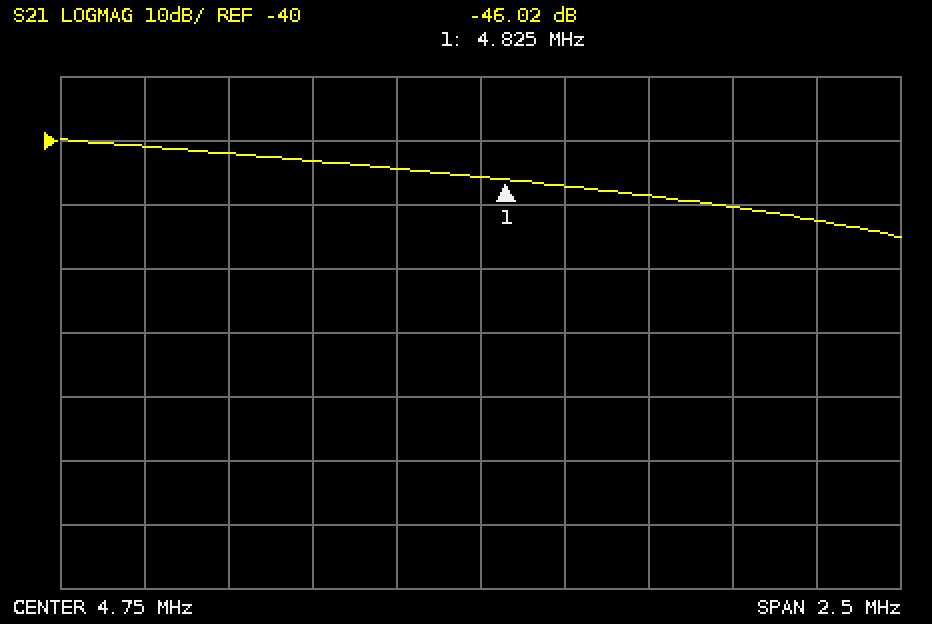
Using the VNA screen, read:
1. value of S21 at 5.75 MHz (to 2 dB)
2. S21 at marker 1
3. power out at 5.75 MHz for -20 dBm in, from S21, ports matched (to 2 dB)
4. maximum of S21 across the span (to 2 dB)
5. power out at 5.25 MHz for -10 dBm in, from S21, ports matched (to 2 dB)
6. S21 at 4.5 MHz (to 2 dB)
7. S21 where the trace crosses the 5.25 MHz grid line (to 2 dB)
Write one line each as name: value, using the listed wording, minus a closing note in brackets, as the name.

value of S21 at 5.75 MHz: -52 dB
S21 at marker 1: -46.02 dB
power out at 5.75 MHz for -20 dBm in, from S21, ports matched: -72 dBm
maximum of S21 across the span: -40 dB
power out at 5.25 MHz for -10 dBm in, from S21, ports matched: -58 dBm
S21 at 4.5 MHz: -44 dB
S21 where the trace crosses the 5.25 MHz grid line: -48 dB
